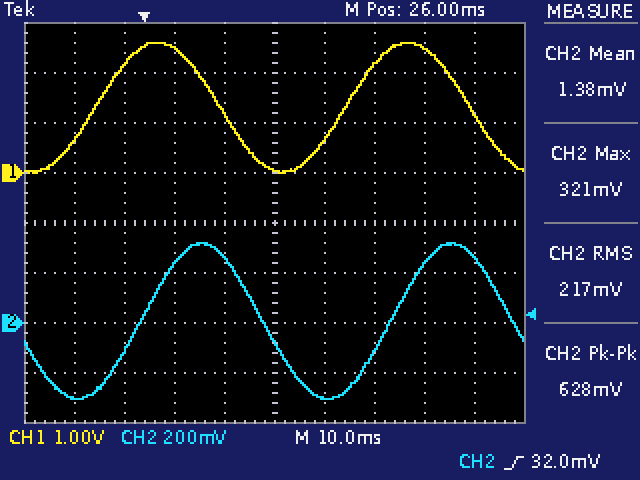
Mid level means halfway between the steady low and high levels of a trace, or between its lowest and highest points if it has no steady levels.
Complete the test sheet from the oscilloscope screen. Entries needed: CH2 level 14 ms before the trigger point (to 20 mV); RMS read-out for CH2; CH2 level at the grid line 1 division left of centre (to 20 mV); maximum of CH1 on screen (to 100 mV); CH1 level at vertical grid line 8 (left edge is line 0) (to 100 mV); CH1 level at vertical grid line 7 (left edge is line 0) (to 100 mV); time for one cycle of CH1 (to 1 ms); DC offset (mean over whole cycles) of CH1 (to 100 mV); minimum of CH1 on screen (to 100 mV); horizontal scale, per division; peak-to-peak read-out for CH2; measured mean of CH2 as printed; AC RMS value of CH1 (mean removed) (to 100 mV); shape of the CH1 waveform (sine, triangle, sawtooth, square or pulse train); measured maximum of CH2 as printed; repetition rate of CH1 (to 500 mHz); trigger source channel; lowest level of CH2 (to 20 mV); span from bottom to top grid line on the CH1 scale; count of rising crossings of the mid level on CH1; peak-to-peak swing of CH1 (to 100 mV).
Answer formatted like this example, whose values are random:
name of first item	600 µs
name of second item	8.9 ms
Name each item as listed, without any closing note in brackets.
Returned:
CH2 level 14 ms before the trigger point	-300 mV
RMS read-out for CH2	217 mV
CH2 level at the grid line 1 division left of centre	260 mV
maximum of CH1 on screen	2.6 V
CH1 level at vertical grid line 8 (left edge is line 0)	2.5 V
CH1 level at vertical grid line 7 (left edge is line 0)	2.2 V
time for one cycle of CH1	50 ms
DC offset (mean over whole cycles) of CH1	1.3 V
minimum of CH1 on screen	0.0 V
horizontal scale, per division	10 ms
peak-to-peak read-out for CH2	628 mV
measured mean of CH2 as printed	1.38 mV
AC RMS value of CH1 (mean removed)	900 mV
shape of the CH1 waveform	sine
measured maximum of CH2 as printed	321 mV
repetition rate of CH1	20.0 Hz
trigger source channel	CH2
lowest level of CH2	-300 mV
span from bottom to top grid line on the CH1 scale	8 V
count of rising crossings of the mid level on CH1	2
peak-to-peak swing of CH1	2.6 V
